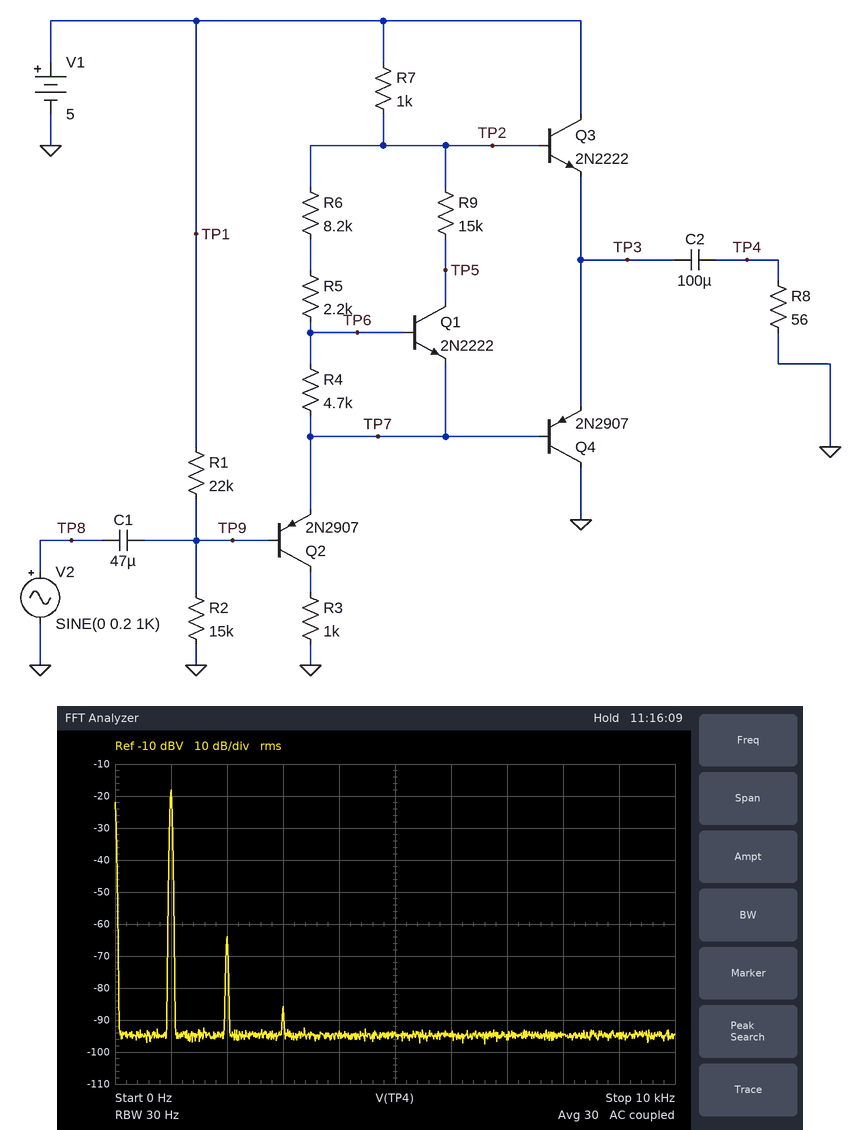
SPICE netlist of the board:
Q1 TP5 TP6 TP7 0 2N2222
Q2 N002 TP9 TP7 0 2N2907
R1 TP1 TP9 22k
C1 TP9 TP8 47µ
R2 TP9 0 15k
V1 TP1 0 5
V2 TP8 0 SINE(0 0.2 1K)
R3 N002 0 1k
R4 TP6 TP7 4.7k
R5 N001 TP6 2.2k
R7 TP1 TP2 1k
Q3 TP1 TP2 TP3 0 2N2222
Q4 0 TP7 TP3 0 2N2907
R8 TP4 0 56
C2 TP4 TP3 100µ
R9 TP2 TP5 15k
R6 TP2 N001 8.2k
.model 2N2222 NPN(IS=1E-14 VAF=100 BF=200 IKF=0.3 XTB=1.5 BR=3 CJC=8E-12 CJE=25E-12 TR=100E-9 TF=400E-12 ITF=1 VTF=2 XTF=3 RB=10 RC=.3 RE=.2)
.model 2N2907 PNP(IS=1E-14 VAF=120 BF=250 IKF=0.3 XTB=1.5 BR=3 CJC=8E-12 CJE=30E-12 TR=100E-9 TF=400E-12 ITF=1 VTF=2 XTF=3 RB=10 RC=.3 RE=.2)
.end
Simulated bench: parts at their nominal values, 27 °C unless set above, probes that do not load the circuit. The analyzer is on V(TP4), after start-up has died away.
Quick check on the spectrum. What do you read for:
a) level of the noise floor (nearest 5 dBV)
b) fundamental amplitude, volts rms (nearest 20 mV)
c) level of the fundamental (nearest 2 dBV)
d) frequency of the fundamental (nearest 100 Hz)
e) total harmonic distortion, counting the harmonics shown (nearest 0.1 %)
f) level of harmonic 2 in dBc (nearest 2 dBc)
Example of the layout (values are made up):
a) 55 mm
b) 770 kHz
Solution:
a) -95 dBV
b) 120 mV
c) -18 dBV
d) 1.0 kHz
e) 0.5 %
f) -46 dBc
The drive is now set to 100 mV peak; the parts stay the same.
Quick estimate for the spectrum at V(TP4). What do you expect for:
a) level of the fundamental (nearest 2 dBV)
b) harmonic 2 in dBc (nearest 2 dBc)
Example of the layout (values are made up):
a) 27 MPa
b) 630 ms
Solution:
a) -24 dBV
b) -52 dBc
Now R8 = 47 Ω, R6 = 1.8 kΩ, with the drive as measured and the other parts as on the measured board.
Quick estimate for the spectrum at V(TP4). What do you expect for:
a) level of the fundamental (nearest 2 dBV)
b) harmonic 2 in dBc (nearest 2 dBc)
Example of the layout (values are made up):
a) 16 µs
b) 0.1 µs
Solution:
a) -18 dBV
b) -42 dBc
